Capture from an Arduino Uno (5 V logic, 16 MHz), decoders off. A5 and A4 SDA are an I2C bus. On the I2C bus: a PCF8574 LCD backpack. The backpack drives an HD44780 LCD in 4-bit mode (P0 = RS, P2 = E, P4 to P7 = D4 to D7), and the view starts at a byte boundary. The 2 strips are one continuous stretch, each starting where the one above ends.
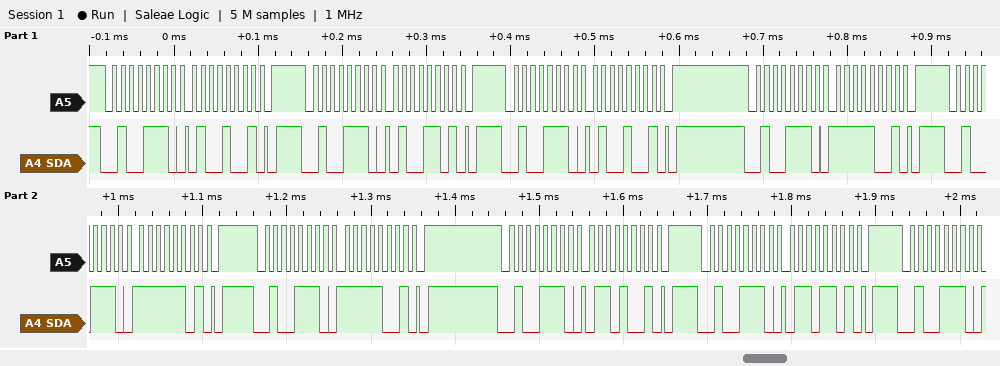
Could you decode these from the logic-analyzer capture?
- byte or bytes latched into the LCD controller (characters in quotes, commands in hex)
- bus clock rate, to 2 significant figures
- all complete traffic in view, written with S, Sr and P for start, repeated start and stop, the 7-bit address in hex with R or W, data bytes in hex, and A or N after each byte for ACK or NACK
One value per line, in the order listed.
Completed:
'O'
100 kHz
S 27W A 49 A P S 27W A 4D A P S 27W A 49 A P S 27W A F9 A P S 27W A FD A P S 27W A F9 A P S 27W A 69 A P S 27W A 6D A P S 27W A
